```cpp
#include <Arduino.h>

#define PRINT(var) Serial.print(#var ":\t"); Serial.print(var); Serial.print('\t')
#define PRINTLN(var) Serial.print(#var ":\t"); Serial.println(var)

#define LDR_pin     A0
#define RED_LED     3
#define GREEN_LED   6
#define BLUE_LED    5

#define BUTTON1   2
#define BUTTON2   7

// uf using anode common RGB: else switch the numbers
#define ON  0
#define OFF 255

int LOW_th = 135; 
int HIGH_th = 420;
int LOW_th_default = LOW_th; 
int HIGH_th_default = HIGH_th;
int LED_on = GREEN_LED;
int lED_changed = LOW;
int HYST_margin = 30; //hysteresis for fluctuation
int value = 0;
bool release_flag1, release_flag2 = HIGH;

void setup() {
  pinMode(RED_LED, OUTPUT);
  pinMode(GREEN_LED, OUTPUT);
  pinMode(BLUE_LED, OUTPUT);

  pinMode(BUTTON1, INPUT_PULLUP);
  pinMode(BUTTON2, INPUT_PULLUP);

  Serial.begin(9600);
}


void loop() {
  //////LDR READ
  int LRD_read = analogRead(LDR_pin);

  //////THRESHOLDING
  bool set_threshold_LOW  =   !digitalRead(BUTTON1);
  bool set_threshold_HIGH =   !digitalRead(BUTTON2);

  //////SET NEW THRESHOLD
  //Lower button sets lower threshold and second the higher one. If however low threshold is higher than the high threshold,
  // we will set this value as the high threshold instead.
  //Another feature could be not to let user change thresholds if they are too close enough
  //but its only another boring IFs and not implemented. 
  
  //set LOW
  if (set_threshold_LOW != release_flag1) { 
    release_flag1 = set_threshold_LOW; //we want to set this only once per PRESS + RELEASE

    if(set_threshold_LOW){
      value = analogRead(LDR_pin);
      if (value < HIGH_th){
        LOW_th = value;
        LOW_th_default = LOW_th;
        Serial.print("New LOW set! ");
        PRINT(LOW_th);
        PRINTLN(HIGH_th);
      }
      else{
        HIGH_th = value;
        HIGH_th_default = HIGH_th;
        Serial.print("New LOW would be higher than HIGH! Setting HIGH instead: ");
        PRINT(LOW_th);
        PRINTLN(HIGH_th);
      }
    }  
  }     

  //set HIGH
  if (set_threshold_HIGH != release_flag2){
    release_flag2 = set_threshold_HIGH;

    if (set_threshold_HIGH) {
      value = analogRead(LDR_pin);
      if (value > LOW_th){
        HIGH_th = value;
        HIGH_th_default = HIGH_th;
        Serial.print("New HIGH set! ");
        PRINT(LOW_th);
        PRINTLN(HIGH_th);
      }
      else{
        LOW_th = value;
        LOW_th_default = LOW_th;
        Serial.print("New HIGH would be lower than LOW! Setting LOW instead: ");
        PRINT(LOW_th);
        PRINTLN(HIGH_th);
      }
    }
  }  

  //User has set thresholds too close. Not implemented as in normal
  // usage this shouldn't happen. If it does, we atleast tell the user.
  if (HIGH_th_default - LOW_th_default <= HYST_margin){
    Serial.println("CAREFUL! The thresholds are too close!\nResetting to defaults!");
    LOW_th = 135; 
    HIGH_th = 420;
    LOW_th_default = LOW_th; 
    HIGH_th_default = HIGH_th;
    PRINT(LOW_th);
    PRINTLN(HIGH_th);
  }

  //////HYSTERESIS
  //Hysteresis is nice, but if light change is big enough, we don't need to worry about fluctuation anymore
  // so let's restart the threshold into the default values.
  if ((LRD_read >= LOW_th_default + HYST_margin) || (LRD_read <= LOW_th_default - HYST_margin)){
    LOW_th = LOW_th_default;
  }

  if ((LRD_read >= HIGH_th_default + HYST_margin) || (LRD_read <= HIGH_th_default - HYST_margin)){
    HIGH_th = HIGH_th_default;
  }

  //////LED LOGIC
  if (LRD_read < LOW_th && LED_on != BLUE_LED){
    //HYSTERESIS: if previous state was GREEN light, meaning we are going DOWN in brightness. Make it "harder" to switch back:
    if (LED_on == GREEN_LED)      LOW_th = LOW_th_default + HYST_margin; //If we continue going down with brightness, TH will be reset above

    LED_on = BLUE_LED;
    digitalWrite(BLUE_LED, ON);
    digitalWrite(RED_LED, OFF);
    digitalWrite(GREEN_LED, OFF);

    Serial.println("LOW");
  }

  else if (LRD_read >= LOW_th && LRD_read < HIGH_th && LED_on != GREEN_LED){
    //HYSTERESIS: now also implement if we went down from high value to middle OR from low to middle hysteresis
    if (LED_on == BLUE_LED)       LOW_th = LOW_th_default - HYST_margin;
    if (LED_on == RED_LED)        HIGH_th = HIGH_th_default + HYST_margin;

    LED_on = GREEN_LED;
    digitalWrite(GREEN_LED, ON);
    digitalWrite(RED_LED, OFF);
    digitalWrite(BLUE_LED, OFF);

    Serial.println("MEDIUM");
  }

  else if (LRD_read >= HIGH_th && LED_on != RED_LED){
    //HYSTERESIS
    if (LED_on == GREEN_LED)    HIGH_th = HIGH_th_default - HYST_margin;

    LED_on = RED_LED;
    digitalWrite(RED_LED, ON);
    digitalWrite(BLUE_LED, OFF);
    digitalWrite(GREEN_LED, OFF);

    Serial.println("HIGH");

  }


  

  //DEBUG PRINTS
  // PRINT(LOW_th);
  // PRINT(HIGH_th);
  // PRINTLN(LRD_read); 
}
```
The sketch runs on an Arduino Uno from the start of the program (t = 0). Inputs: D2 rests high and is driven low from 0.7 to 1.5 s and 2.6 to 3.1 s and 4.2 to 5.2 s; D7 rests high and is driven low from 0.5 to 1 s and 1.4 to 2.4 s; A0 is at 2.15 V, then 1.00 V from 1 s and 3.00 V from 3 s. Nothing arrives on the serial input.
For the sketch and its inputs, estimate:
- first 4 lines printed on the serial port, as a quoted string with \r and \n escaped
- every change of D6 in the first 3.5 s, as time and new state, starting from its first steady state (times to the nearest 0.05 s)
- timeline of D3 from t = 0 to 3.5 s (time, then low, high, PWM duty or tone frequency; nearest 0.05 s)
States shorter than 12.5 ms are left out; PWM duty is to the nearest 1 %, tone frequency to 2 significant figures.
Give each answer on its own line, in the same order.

"HIGH\r\nNew HIGH set! LOW_th:\t135\tHIGH_th:\t440\r\nNew LOW would be higher than HIGH! Setting HIGH instead: LOW_th:\t135\tHIGH_th:\t440\r\nMEDIUM\r\n"
0 s high; 1 s low; 1.4 s high
0 s low; 1 s high; 1.4 s low
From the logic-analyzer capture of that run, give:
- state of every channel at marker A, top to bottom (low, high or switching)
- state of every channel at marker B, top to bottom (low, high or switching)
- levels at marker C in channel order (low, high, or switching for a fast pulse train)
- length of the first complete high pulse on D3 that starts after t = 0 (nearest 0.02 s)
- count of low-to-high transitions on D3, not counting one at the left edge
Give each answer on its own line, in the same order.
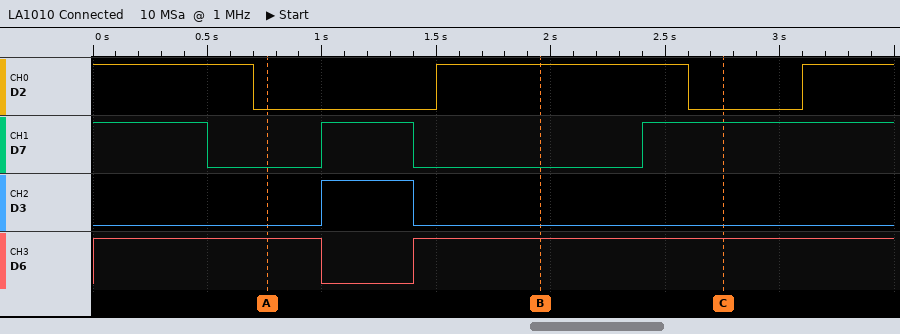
D2 low, D7 low, D3 low, D6 high
D2 high, D7 low, D3 low, D6 high
D2 low, D7 high, D3 low, D6 high
0.40 s
1
